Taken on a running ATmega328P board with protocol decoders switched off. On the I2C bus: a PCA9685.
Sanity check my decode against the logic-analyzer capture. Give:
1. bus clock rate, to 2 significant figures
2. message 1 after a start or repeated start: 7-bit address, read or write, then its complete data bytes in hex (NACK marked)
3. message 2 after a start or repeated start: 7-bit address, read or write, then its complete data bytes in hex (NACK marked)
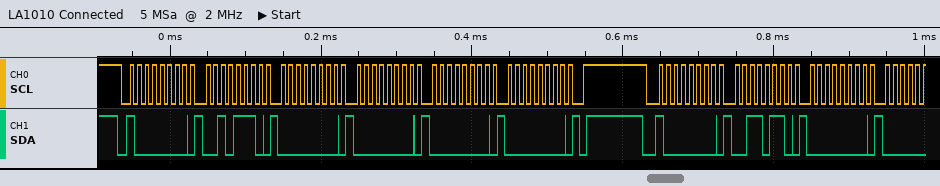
100 kHz
0x40 write: 2E 00 00 00 00
0x40 write: 36 00
